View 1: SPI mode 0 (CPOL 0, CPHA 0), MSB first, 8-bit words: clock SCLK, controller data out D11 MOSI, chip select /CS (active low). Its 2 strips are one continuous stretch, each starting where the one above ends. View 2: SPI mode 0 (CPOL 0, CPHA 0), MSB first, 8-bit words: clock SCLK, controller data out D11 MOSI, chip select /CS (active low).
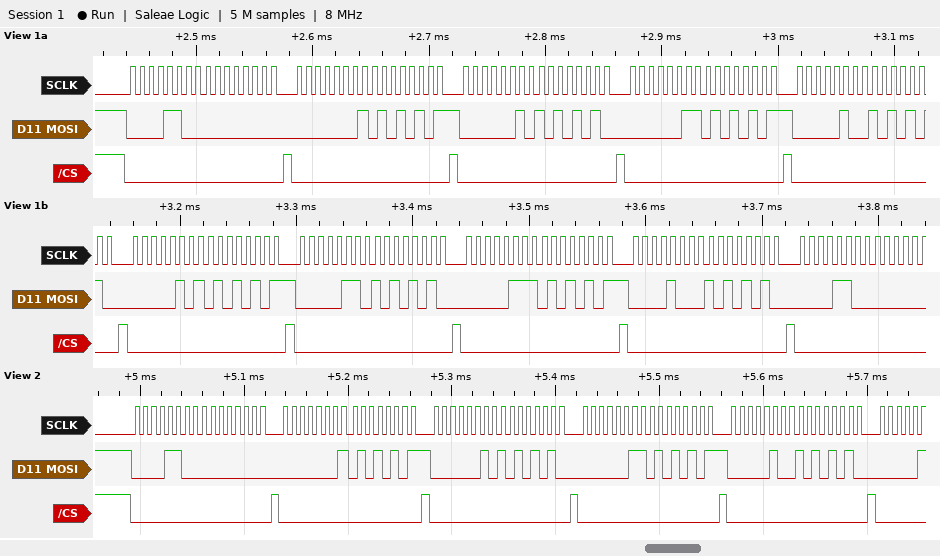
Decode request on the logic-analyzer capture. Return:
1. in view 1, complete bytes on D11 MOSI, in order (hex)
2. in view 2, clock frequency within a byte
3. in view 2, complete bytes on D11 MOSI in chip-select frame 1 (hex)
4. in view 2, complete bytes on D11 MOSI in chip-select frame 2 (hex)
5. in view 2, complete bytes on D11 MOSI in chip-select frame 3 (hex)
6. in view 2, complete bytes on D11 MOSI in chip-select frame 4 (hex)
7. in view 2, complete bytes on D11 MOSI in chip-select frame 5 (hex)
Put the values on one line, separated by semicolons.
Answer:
0C 00 01 55 02 AA 03 55 04 AA 05 55 06 AA 07 55 08 AA 0C; 125 kHz; 0C 00; 01 55; 02 AA; 03 55; 04 AA
